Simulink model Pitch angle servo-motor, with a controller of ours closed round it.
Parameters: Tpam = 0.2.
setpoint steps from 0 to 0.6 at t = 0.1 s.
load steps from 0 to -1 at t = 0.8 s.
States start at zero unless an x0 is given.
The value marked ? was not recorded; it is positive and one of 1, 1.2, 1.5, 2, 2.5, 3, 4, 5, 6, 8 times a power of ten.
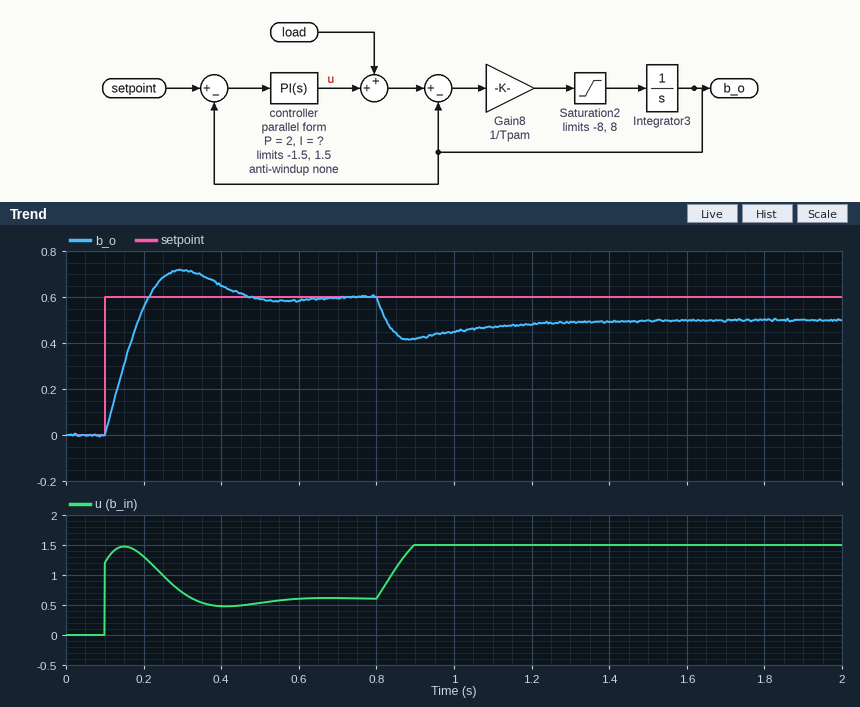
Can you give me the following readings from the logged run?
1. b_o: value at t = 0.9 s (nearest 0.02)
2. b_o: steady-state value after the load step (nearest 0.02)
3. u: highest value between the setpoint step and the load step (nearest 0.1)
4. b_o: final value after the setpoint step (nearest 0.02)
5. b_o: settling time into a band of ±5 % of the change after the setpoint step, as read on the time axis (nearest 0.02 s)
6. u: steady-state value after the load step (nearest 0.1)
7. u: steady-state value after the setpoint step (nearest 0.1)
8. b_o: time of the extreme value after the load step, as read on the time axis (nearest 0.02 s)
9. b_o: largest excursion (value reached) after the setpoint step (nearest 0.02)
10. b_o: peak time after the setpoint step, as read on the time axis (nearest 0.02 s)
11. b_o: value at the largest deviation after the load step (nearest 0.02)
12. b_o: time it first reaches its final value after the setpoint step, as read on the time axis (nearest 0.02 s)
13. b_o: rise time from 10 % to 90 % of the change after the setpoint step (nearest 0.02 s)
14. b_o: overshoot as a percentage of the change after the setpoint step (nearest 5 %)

0.42
0.50
1.5
0.60
0.42 s
1.5
0.6
0.88 s
0.72
0.30 s
0.42
0.22 s
0.08 s
20 %
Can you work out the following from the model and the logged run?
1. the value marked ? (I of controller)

40
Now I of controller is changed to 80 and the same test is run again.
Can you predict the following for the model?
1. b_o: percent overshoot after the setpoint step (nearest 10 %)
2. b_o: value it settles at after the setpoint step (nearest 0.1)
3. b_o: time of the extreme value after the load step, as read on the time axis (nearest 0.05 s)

40 %
0.6
0.85 s
